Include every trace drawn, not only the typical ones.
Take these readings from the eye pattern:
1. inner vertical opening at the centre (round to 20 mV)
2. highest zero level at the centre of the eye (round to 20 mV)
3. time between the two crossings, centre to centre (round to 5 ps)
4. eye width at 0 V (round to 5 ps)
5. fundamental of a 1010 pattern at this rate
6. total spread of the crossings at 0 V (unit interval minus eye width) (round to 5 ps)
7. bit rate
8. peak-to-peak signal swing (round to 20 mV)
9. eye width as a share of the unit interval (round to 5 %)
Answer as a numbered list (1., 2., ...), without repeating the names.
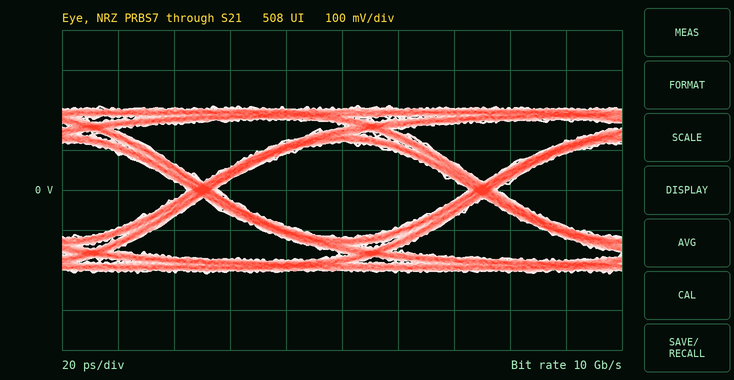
1. 240 mV
2. -120 mV
3. 100 ps
4. 90 ps
5. 5 GHz
6. 10 ps
7. 10 Gb/s
8. 420 mV
9. 90 %
